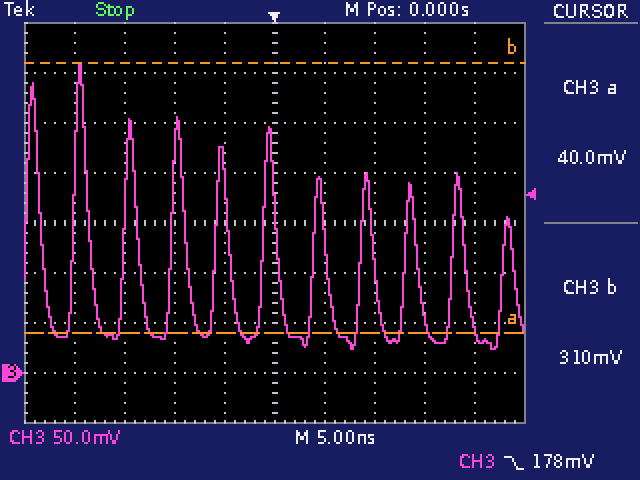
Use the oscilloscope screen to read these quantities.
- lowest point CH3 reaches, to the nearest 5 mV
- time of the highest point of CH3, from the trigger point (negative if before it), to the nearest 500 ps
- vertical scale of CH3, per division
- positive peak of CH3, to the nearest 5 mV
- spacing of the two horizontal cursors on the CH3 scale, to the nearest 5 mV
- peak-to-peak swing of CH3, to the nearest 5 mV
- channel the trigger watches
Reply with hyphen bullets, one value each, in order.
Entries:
- 25 mV
- -19.5 ns
- 50 mV
- 310 mV
- 270 mV
- 285 mV
- CH3
